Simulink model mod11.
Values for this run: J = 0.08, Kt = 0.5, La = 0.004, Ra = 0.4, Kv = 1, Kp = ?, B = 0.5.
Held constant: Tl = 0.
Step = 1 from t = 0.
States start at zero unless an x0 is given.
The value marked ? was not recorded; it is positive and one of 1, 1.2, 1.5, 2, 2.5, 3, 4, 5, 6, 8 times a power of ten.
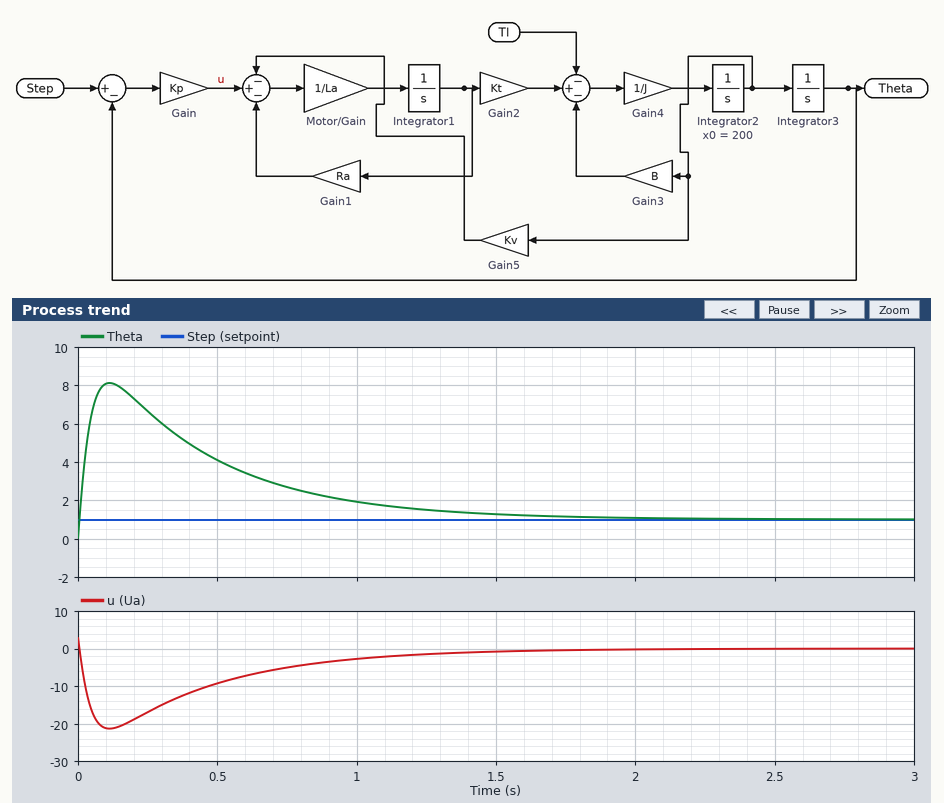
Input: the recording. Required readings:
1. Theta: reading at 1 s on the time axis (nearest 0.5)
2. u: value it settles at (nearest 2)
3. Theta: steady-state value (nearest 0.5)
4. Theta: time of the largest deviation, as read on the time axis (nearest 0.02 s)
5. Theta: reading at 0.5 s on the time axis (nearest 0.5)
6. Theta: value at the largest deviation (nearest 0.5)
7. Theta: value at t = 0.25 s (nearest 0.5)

2.0
0
1.0
0.12 s
4.0
8.0
6.5
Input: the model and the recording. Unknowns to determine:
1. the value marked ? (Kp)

3
